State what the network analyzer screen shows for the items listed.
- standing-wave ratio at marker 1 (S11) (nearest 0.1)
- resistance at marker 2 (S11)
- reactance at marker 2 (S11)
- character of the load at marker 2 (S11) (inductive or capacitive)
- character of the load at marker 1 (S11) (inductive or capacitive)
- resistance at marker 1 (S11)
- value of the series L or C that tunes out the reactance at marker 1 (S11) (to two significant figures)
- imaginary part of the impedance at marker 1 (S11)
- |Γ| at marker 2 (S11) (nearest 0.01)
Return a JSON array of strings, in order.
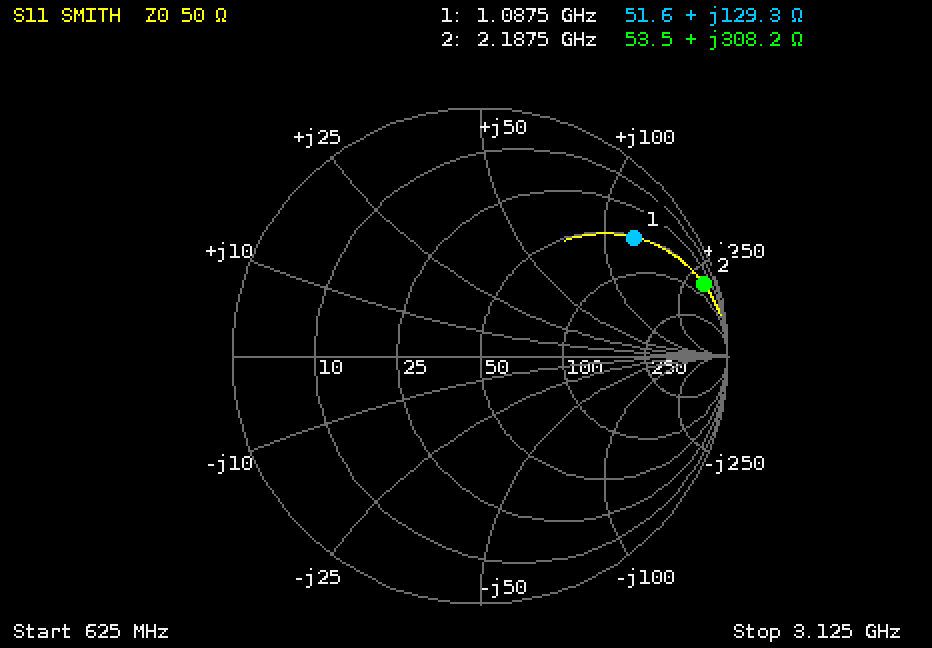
["8.4", "53.5 Ω", "+308.2 Ω", "inductive", "inductive", "51.6 Ω", "1.1 pF", "+129.3 Ω", "0.95"]
